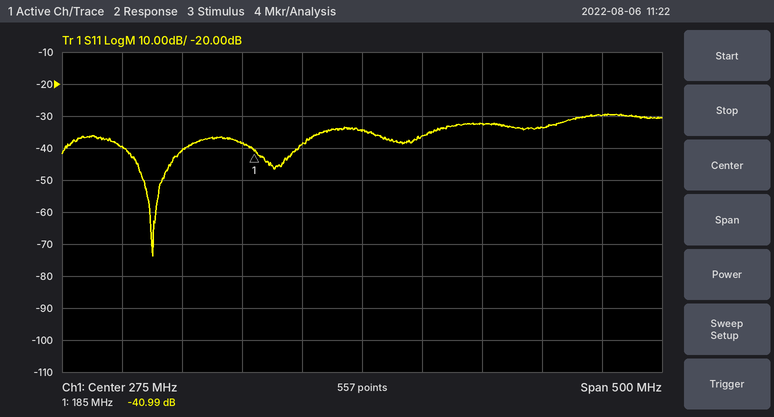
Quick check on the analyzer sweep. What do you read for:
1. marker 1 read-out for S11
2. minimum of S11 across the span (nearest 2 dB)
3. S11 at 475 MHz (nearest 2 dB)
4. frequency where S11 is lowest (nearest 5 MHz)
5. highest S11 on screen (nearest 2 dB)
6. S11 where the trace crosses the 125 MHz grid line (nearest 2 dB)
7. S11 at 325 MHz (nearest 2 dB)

-40.99 dB
-74 dB
-30 dB
100 MHz
-30 dB
-40 dB
-36 dB
